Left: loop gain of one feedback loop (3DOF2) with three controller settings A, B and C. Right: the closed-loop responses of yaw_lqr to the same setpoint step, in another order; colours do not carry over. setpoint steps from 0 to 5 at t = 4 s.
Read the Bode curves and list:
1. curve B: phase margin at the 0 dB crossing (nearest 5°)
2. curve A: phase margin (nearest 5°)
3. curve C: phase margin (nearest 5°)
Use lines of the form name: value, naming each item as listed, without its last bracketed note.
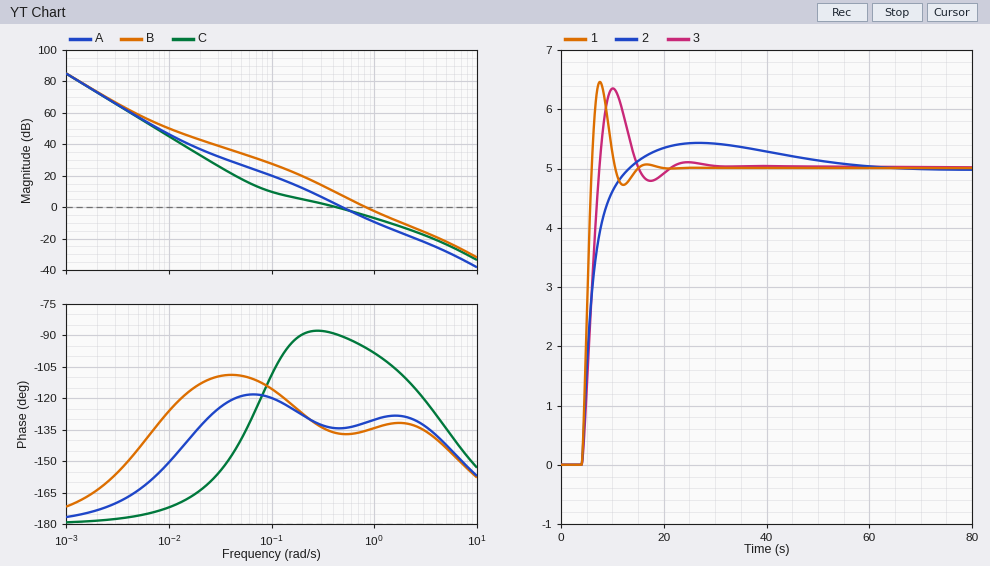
curve B: phase margin at the 0 dB crossing: 45°
curve A: phase margin: 45°
curve C: phase margin: 90°
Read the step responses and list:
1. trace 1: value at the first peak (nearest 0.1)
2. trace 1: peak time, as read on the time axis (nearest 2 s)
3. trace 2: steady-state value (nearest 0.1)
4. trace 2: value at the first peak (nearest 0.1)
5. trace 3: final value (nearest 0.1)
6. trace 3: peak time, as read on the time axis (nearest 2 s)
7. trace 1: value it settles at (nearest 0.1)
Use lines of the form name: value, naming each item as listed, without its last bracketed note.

trace 1: value at the first peak: 6.5
trace 1: peak time, as read on the time axis: 8 s
trace 2: steady-state value: 5.0
trace 2: value at the first peak: 5.4
trace 3: final value: 5.0
trace 3: peak time, as read on the time axis: 10 s
trace 1: value it settles at: 5.0
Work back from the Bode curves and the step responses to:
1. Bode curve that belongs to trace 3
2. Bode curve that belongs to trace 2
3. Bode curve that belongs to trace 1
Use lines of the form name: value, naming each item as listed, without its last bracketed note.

Bode curve that belongs to trace 3: A
Bode curve that belongs to trace 2: C
Bode curve that belongs to trace 1: B
